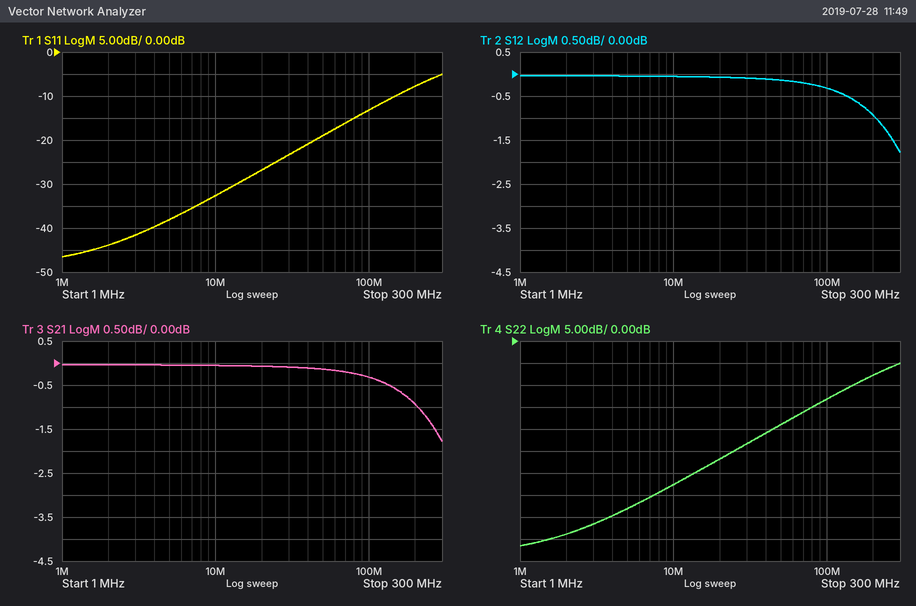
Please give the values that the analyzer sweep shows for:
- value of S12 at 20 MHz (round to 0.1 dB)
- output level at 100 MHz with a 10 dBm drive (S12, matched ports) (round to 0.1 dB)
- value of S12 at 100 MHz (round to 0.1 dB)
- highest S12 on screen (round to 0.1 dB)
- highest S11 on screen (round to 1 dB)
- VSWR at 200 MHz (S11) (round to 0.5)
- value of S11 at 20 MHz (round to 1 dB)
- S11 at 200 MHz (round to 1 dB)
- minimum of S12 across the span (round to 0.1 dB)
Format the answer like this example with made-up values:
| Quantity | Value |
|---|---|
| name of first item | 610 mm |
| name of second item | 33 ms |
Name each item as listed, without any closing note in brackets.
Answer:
| Quantity | Value |
|---|---|
| value of S12 at 20 MHz | -0.1 dB |
| output level at 100 MHz with a 10 dBm drive (S12, matched ports) | 9.7 dBm |
| value of S12 at 100 MHz | -0.3 dB |
| highest S12 on screen | 0.0 dB |
| highest S11 on screen | -5 dB |
| VSWR at 200 MHz (S11) | 2.5 |
| value of S11 at 20 MHz | -27 dB |
| S11 at 200 MHz | -8 dB |
| minimum of S12 across the span | -1.8 dB |
